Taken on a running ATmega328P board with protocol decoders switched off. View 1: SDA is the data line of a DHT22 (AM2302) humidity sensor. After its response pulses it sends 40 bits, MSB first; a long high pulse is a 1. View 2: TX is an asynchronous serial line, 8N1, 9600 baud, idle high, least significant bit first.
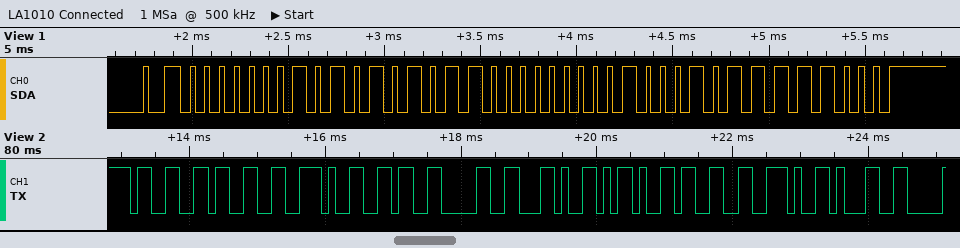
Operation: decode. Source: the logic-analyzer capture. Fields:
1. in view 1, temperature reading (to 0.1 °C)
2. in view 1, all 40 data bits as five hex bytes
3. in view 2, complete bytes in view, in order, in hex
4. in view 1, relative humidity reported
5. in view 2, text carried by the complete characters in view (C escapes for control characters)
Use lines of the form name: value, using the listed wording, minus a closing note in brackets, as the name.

in view 1, temperature reading: -3.4 °C
in view 1, all 40 data bits as five hex bytes: 01 55 80 22 F8
in view 2, complete bytes in view, in order, in hex: 33 33 2E 36 30 2C 2D 33 2E 31
in view 1, relative humidity reported: 34.1 %
in view 2, text carried by the complete characters in view: "33.60,-3.1"
